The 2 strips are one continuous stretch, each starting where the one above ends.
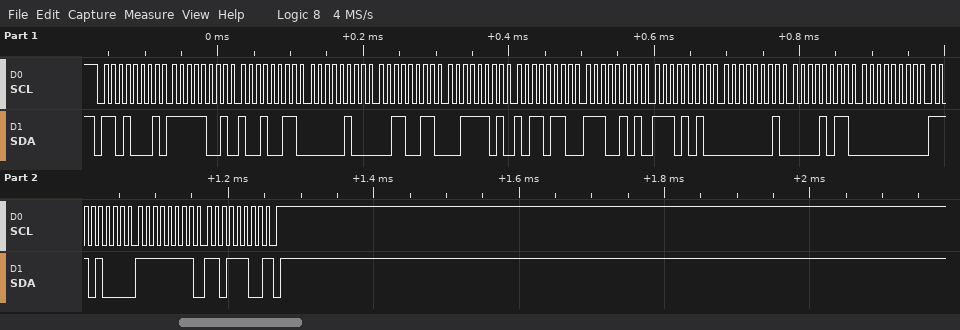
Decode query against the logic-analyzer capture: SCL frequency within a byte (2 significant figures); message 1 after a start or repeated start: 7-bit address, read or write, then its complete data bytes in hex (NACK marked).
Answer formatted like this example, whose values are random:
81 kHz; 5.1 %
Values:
100 kHz; 0x68 read: F9 93 04 33 3D B6 E5 EA 01 0B 00 E8 FF DC NACK
